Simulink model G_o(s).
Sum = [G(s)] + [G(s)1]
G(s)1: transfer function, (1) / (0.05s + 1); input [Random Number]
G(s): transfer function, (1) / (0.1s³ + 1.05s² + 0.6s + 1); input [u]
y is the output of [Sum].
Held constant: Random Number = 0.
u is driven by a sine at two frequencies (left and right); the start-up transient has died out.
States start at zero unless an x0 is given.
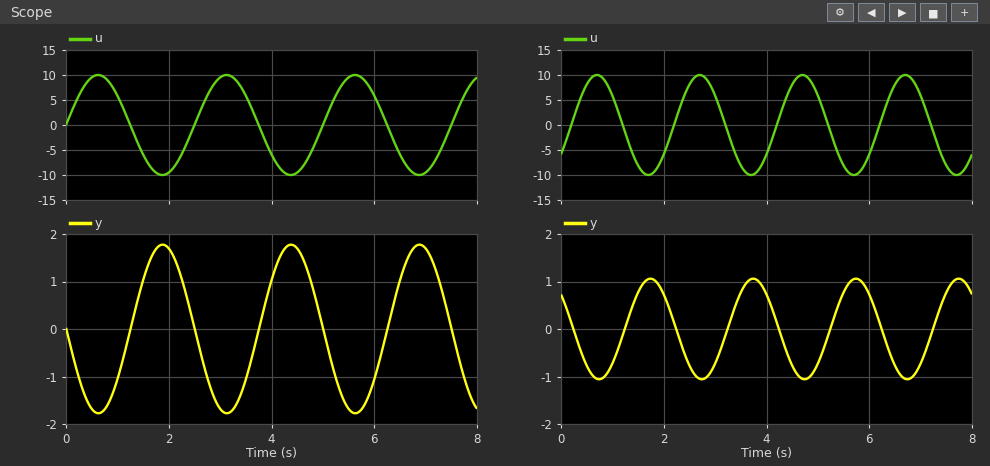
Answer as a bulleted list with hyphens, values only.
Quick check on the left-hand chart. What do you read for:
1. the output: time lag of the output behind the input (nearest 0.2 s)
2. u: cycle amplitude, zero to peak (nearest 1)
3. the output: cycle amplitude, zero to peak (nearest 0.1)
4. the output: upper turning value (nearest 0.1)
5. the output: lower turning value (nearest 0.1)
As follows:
- 1.2 s
- 10
- 1.8
- 1.8
- -1.8
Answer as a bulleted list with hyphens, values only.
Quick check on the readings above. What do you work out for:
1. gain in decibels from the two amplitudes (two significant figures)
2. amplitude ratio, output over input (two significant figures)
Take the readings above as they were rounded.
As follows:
- -15 dB
- 0.18
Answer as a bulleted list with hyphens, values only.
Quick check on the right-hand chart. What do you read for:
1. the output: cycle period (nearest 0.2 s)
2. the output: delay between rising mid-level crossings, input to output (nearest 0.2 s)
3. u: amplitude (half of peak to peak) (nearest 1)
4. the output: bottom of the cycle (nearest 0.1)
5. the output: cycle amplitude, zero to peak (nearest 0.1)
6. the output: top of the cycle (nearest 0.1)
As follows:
- 2.0 s
- 1.0 s
- 10
- -1.1
- 1.1
- 1.1
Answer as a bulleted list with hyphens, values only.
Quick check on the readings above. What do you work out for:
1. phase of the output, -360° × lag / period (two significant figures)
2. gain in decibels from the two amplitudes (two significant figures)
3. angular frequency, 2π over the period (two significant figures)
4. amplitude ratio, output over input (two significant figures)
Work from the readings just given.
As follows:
- -180°
- -19 dB
- 3.1 rad/s
- 0.11
